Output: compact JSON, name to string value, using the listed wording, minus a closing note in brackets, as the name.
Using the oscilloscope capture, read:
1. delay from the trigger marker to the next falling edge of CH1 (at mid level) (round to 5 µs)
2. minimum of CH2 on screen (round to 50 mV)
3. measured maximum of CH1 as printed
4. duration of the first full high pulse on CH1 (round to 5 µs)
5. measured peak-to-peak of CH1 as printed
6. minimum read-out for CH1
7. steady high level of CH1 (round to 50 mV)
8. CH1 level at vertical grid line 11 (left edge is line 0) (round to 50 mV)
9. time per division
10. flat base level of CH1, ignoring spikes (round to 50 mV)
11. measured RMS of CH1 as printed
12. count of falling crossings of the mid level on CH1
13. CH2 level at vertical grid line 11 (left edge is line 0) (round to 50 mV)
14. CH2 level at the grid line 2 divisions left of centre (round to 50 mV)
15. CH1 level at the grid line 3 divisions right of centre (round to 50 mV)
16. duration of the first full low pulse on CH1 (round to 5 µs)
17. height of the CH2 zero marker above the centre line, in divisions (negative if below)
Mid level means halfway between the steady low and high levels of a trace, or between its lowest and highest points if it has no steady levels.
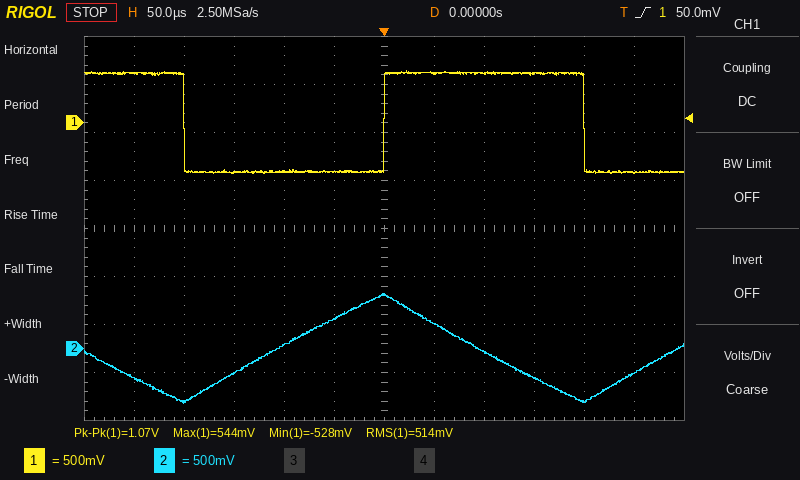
{"delay from the trigger marker to the next falling edge of CH1 (at mid level)": "200 µs", "minimum of CH2 on screen": "-550 mV", "measured maximum of CH1 as printed": "544 mV", "duration of the first full high pulse on CH1": "200 µs", "measured peak-to-peak of CH1 as printed": "1.07 V", "minimum read-out for CH1": "-528 mV", "steady high level of CH1": "500 mV", "CH1 level at vertical grid line 11 (left edge is line 0)": "-500 mV", "time per division": "50 µs", "flat base level of CH1, ignoring spikes": "-500 mV", "measured RMS of CH1 as printed": "514 mV", "count of falling crossings of the mid level on CH1": "2", "CH2 level at vertical grid line 11 (left edge is line 0)": "-250 mV", "CH2 level at the grid line 2 divisions left of centre": "50 mV", "CH1 level at the grid line 3 divisions right of centre": "500 mV", "duration of the first full low pulse on CH1": "200 µs", "height of the CH2 zero marker above the centre line, in divisions": "-2.5 div"}
